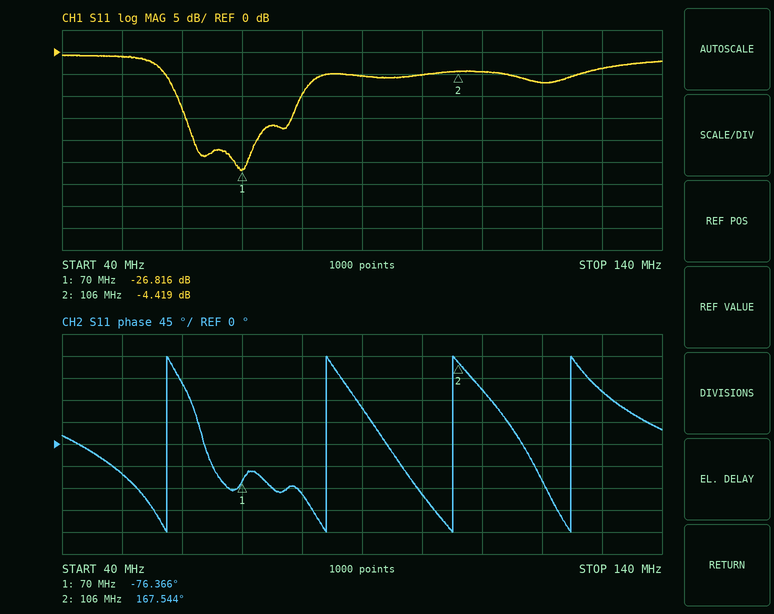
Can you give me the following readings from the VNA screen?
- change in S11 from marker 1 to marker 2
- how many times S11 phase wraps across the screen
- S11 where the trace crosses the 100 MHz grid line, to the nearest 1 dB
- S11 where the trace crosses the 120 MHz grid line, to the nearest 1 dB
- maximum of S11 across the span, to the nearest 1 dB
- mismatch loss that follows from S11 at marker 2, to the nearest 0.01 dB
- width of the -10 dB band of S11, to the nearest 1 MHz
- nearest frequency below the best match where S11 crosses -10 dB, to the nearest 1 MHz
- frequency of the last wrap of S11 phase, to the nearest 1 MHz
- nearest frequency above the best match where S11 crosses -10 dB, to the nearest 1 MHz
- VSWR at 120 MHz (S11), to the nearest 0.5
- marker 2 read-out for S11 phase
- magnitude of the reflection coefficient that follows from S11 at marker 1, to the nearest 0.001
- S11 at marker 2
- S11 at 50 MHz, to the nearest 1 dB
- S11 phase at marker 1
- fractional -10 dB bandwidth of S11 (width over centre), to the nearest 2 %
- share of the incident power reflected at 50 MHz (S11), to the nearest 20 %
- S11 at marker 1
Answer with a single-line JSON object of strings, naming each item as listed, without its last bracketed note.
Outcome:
{"change in S11 from marker 1 to marker 2": "22.397 dB", "how many times S11 phase wraps across the screen": "4", "S11 where the trace crosses the 100 MHz grid line, to the nearest 1 dB": "-5 dB", "S11 where the trace crosses the 120 MHz grid line, to the nearest 1 dB": "-7 dB", "maximum of S11 across the span, to the nearest 1 dB": "-1 dB", "mismatch loss that follows from S11 at marker 2, to the nearest 0.01 dB": "1.95 dB", "width of the -10 dB band of S11, to the nearest 1 MHz": "21 MHz", "nearest frequency below the best match where S11 crosses -10 dB, to the nearest 1 MHz": "59 MHz", "frequency of the last wrap of S11 phase, to the nearest 1 MHz": "125 MHz", "nearest frequency above the best match where S11 crosses -10 dB, to the nearest 1 MHz": "80 MHz", "VSWR at 120 MHz (S11), to the nearest 0.5": "2.5", "marker 2 read-out for S11 phase": "167.544°", "magnitude of the reflection coefficient that follows from S11 at marker 1, to the nearest 0.001": "0.046", "S11 at marker 2": "-4.419 dB", "S11 at 50 MHz, to the nearest 1 dB": "-1 dB", "S11 phase at marker 1": "-76.366°", "fractional -10 dB bandwidth of S11 (width over centre), to the nearest 2 %": "30 %", "share of the incident power reflected at 50 MHz (S11), to the nearest 20 %": "80 %", "S11 at marker 1": "-26.816 dB"}
